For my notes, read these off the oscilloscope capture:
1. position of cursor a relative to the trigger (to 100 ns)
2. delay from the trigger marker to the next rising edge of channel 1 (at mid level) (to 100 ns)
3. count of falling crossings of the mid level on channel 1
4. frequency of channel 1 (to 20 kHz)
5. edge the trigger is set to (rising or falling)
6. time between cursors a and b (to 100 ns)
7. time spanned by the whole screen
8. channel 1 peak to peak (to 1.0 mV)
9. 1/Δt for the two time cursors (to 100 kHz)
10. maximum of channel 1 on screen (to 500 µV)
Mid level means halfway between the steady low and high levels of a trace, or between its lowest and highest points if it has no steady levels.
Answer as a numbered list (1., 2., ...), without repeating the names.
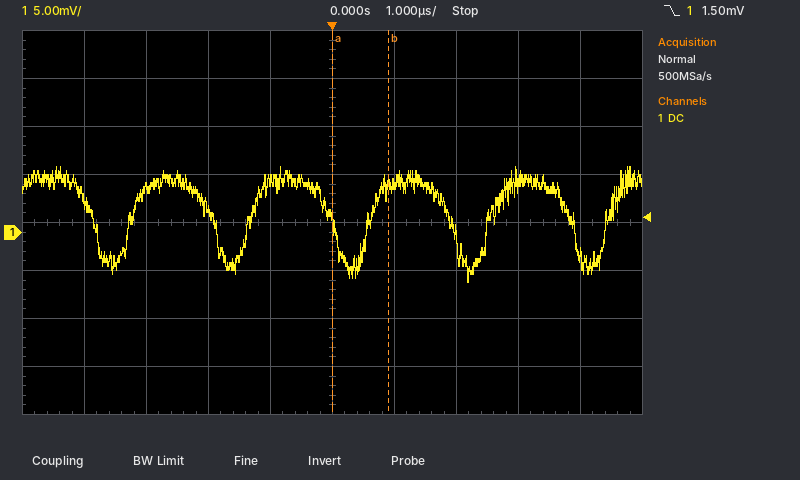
1. 0.0 µs
2. 600 ns
3. 5
4. 520 kHz
5. falling
6. 900 ns
7. 10 µs
8. 12.0 mV
9. 1.1 MHz
10. 7.0 mV
